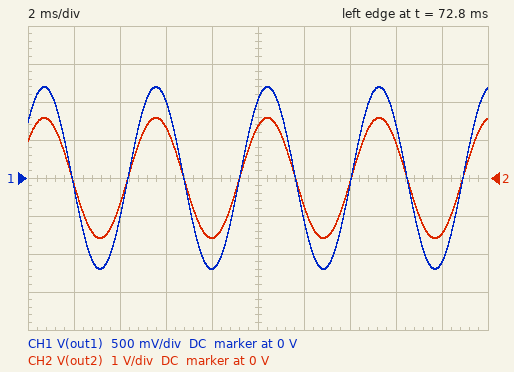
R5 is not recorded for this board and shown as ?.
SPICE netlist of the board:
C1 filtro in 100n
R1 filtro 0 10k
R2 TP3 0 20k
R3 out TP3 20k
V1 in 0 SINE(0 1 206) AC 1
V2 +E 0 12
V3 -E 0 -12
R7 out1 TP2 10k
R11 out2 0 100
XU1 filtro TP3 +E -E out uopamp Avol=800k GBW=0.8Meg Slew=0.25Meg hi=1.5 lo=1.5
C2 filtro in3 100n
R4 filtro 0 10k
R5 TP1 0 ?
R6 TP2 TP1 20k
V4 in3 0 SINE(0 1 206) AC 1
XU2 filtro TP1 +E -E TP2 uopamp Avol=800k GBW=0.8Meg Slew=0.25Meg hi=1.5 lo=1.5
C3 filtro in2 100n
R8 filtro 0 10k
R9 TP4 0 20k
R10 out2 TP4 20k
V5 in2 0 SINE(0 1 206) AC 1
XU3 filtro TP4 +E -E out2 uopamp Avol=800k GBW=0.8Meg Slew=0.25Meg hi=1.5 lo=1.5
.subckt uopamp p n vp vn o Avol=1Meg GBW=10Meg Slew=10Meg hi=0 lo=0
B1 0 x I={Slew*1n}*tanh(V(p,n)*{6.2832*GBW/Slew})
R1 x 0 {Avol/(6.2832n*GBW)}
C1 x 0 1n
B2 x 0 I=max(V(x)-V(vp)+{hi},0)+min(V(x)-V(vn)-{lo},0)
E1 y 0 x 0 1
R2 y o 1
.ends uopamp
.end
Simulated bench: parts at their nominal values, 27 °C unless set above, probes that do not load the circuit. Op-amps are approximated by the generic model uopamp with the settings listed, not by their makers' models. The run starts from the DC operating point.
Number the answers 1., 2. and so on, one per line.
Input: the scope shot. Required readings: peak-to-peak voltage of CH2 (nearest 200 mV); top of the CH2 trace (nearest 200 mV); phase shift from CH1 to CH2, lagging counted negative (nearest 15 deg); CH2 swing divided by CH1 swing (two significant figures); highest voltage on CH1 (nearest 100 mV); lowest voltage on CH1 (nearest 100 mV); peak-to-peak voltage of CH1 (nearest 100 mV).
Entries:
1. 3.2 V
2. 1.6 V
3. 0 deg
4. 1.3
5. 1.2 V
6. -1.2 V
7. 2.4 V
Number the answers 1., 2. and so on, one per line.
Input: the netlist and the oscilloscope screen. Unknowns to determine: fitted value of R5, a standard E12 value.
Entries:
1. 39 kΩ
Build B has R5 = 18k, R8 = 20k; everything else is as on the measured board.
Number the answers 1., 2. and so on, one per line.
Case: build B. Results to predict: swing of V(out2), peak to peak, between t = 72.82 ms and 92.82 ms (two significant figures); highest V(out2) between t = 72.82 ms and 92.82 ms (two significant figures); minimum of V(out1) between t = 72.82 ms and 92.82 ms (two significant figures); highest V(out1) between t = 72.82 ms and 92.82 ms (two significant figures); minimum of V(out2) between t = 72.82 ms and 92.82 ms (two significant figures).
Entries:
1. 3.4 V
2. 1.7 V
3. -1.8 V
4. 1.8 V
5. -1.7 V
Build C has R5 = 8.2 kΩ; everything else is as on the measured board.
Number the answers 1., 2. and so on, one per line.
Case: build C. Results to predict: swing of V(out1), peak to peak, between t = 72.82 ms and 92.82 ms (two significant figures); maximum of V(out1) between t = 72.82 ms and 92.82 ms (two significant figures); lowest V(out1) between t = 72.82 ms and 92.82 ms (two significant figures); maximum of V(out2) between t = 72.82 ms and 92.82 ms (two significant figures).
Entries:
1. 5.4 V
2. 2.7 V
3. -2.7 V
4. 1.6 V
